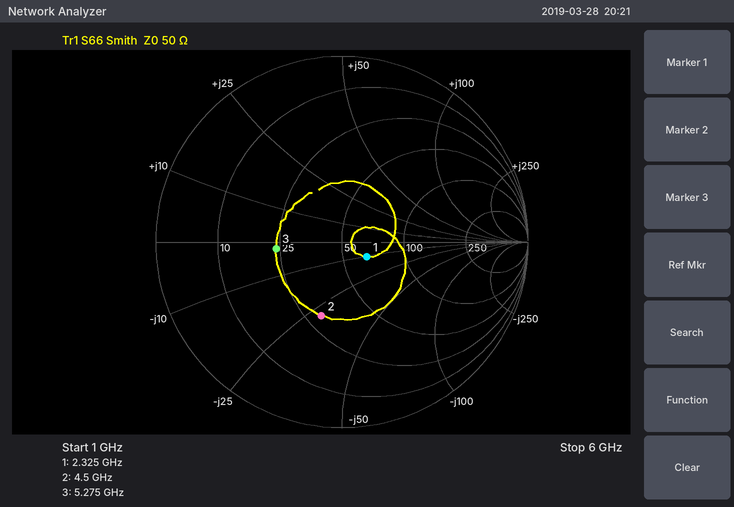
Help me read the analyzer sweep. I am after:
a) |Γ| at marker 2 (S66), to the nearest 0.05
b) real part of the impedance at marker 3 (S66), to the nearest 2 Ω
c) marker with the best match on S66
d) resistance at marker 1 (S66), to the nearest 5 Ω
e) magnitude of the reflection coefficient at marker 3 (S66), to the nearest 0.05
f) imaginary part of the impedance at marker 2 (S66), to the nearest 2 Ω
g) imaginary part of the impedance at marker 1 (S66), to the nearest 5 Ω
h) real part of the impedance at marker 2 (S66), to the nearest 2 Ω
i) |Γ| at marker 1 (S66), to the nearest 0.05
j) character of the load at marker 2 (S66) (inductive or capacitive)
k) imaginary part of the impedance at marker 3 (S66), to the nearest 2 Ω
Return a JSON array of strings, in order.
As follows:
["0.40", "24 Ω", "marker 1", "65 Ω", "0.35", "-28 Ω", "-10 Ω", "30 Ω", "0.15", "capacitive", "-2 Ω"]
